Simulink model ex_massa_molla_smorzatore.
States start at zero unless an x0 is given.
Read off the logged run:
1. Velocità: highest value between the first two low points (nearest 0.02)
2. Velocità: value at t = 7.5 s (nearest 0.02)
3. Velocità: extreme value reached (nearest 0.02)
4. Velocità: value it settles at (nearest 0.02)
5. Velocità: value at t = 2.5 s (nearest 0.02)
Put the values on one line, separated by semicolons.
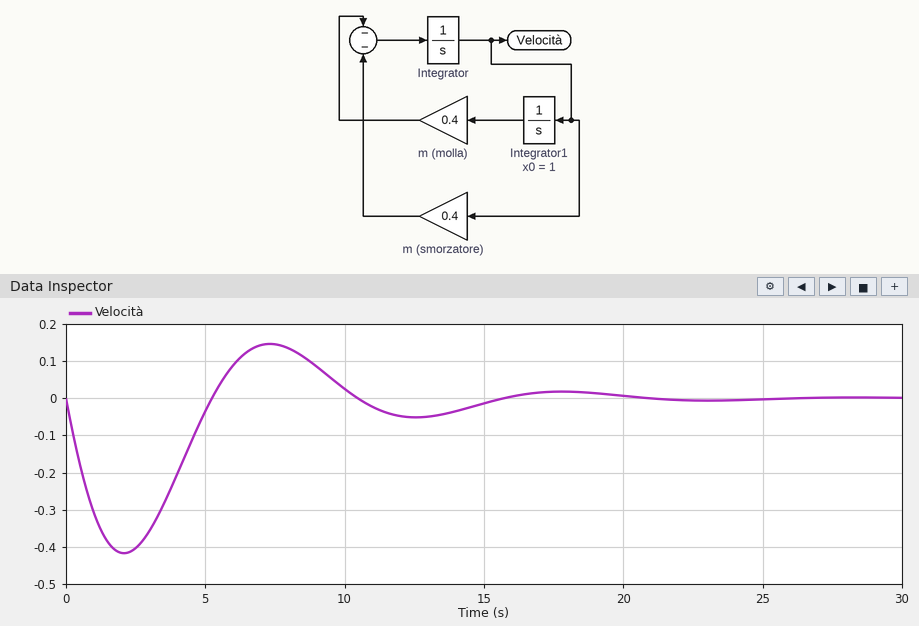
0.14; 0.14; -0.42; 0.00; -0.40
